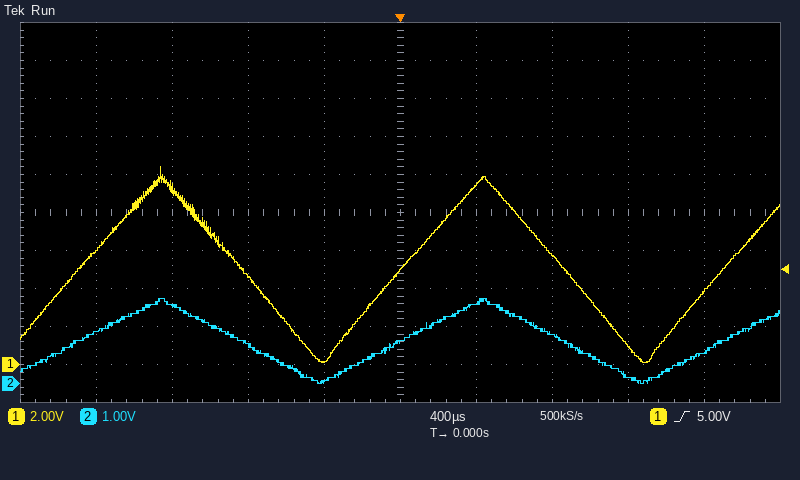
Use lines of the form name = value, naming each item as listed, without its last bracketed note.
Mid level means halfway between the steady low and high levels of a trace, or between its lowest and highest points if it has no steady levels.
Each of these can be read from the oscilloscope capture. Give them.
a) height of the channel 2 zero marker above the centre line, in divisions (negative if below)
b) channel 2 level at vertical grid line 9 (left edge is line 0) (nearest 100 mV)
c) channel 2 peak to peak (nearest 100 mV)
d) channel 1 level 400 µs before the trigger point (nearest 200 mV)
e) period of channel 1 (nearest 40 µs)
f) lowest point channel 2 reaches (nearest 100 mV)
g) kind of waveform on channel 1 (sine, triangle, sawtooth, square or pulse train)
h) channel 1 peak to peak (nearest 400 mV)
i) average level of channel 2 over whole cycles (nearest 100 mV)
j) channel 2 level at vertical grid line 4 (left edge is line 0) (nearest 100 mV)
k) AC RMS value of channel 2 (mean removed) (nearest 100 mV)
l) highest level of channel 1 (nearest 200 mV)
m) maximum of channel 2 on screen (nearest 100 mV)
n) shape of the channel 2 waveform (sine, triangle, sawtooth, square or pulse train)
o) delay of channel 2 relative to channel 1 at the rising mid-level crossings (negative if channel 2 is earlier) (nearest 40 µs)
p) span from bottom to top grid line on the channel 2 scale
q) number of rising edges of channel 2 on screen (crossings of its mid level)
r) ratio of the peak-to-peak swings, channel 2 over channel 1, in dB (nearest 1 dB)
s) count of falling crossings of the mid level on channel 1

height of the channel 2 zero marker above the centre line, in divisions = -4.5 div
channel 2 level at vertical grid line 9 (left edge is line 0) = 900 mV
channel 2 peak to peak = 2.2 V
channel 1 level 400 µs before the trigger point = 200 mV
period of channel 1 = 1.68 ms
lowest point channel 2 reaches = 0.0 V
kind of waveform on channel 1 = triangle
channel 1 peak to peak = 10.4 V
average level of channel 2 over whole cycles = 1.1 V
channel 2 level at vertical grid line 4 (left edge is line 0) = 100 mV
AC RMS value of channel 2 (mean removed) = 600 mV
highest level of channel 1 = 10.4 V
maximum of channel 2 on screen = 2.2 V
shape of the channel 2 waveform = triangle
delay of channel 2 relative to channel 1 at the rising mid-level crossings (negative if channel 2 is earlier) = -40 µs
span from bottom to top grid line on the channel 2 scale = 10 V
number of rising edges of channel 2 on screen = 3
ratio of the peak-to-peak swings, channel 2 over channel 1, in dB = -13 dB
count of falling crossings of the mid level on channel 1 = 2
